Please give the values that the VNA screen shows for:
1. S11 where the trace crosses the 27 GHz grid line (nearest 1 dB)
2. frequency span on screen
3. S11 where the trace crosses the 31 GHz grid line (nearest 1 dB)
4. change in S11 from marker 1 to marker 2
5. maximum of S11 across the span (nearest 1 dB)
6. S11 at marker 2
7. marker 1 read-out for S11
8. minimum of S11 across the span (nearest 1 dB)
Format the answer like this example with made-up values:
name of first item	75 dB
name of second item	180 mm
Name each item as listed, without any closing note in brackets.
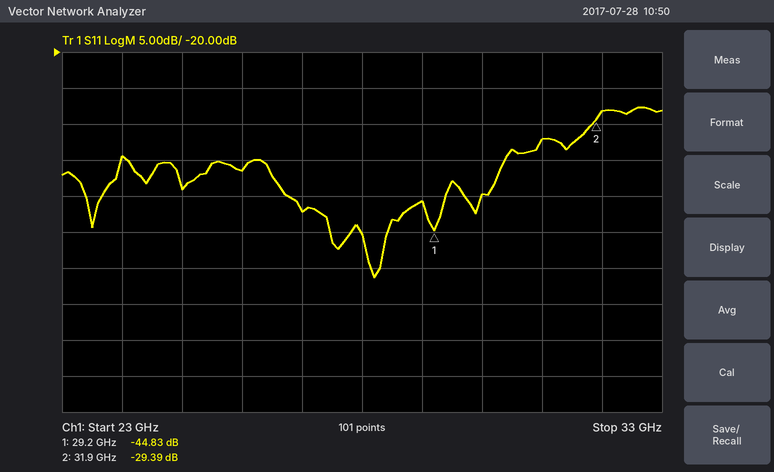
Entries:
S11 where the trace crosses the 27 GHz grid line	-42 dB
frequency span on screen	10 GHz
S11 where the trace crosses the 31 GHz grid line	-32 dB
change in S11 from marker 1 to marker 2	15.44 dB
maximum of S11 across the span	-28 dB
S11 at marker 2	-29.39 dB
marker 1 read-out for S11	-44.83 dB
minimum of S11 across the span	-51 dB
